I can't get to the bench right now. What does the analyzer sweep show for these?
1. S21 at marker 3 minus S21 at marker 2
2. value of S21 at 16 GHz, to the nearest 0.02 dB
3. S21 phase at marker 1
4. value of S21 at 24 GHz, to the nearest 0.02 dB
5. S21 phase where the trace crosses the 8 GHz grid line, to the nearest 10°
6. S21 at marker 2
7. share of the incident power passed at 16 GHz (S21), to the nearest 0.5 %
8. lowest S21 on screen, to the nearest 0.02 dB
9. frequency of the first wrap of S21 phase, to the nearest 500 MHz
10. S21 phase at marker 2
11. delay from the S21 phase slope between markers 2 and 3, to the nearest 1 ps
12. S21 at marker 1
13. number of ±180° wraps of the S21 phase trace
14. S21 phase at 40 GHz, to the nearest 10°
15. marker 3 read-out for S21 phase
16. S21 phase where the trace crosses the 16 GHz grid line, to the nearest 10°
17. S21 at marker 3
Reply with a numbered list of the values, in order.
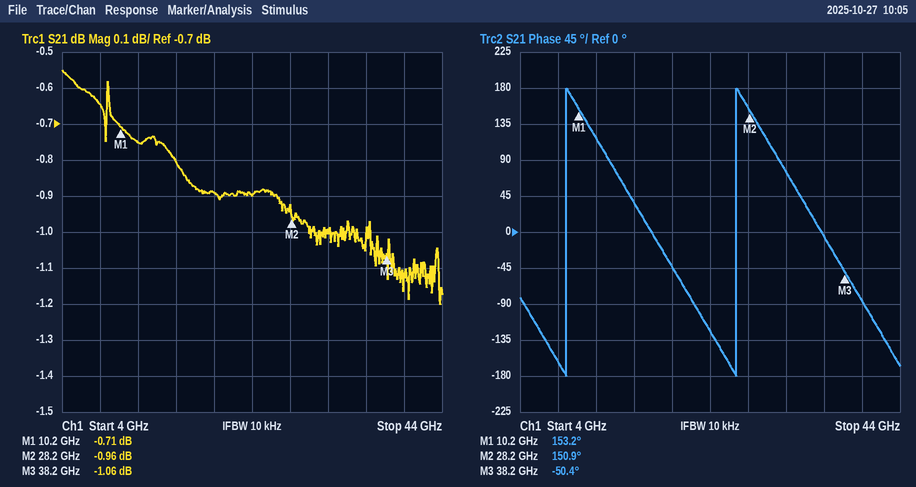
1. -0.10 dB
2. -0.80 dB
3. 153.2°
4. -0.90 dB
5. -160°
6. -0.96 dB
7. 83.0 %
8. -1.20 dB
9. 9.0 GHz
10. 150.9°
11. 56 ps
12. -0.71 dB
13. 2
14. -90°
15. -50.4°
16. 40°
17. -1.06 dB
